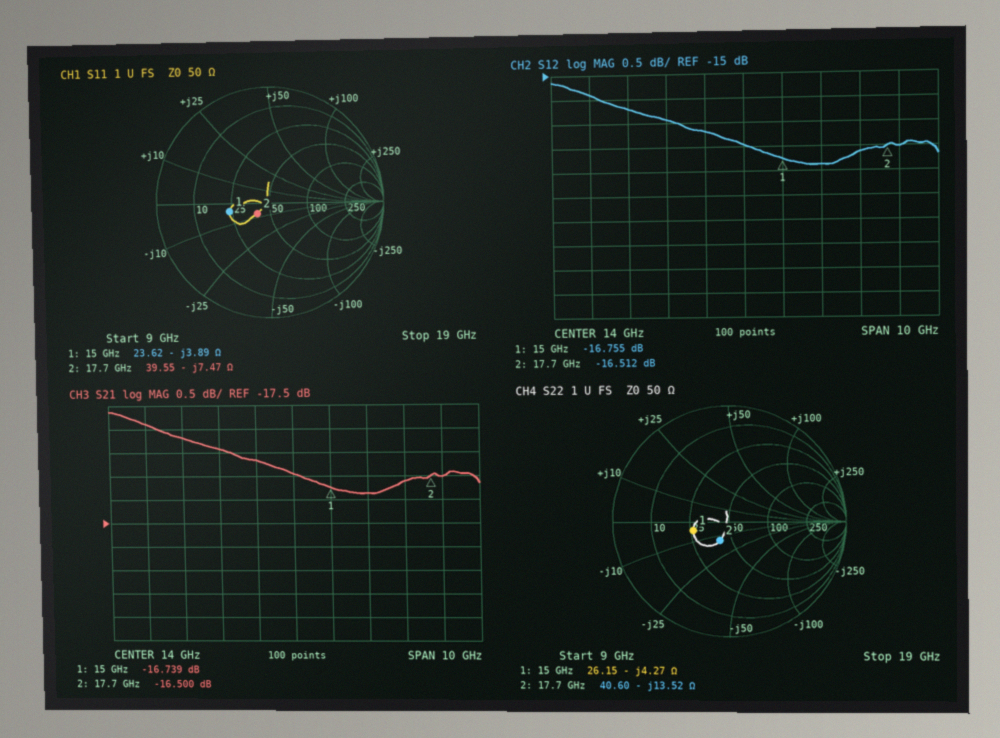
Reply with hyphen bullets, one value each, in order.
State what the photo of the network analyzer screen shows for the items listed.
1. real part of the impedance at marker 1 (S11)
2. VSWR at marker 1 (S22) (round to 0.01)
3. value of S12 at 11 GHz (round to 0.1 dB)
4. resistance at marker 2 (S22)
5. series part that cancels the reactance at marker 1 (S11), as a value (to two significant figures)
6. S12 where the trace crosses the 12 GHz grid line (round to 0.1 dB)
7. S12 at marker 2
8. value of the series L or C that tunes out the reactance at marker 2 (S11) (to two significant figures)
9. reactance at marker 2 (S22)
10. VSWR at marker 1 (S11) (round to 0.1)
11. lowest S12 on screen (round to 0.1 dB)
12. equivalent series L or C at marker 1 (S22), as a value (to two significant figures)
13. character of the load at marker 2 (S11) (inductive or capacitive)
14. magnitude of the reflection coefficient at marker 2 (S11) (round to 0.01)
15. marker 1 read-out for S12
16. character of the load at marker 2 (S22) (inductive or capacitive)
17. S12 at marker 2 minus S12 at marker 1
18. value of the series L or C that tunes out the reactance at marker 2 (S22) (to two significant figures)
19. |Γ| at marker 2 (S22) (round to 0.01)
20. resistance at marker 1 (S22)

- 23.62 Ω
- 1.93
- -15.7 dB
- 40.60 Ω
- 41 pH
- -15.9 dB
- -16.512 dB
- 67 pH
- -13.52 Ω
- 2.1
- -16.9 dB
- 2.5 pF
- capacitive
- 0.14
- -16.755 dB
- capacitive
- 0.243 dB
- 120 pH
- 0.18
- 26.15 Ω
